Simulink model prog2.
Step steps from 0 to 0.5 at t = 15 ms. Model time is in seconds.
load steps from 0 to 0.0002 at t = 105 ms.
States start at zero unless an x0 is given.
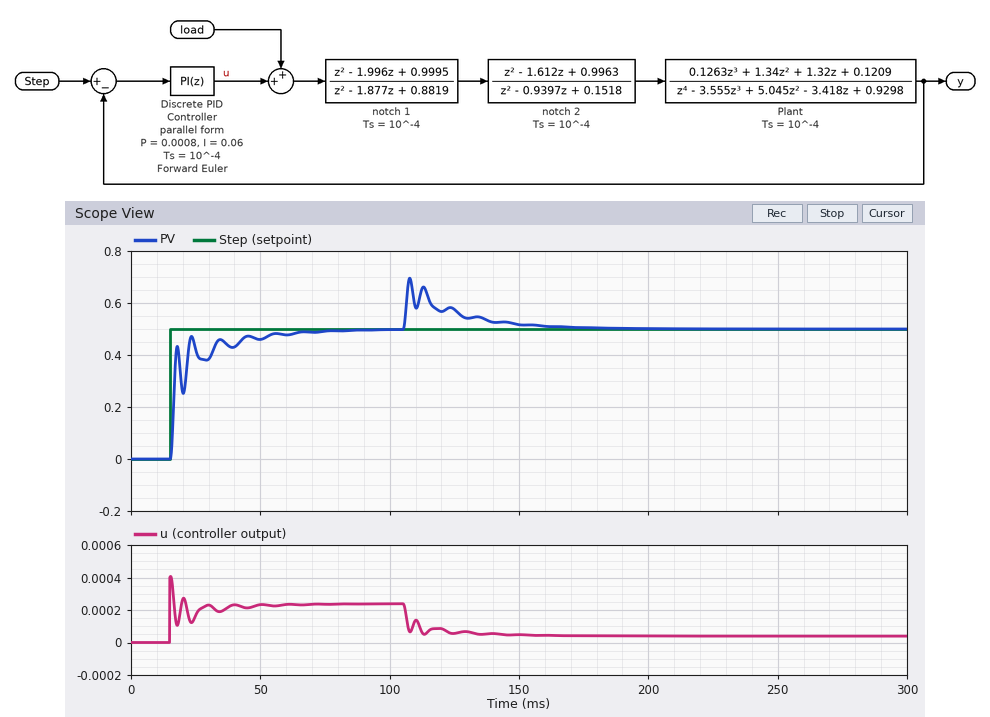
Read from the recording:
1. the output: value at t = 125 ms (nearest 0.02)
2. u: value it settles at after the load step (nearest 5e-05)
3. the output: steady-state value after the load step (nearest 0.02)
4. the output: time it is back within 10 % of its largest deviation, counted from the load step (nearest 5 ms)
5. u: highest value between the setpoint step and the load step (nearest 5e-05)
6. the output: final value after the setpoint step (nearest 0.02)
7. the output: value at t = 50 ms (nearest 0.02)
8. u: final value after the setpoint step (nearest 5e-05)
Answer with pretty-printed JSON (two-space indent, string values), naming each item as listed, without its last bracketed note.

{
  "the output: value at t = 125 ms": "0.58",
  "u: value it settles at after the load step": "0.00005",
  "the output: steady-state value after the load step": "0.50",
  "the output: time it is back within 10 % of its largest deviation, counted from the load step": "45 ms",
  "u: highest value between the setpoint step and the load step": "0.00040",
  "the output: final value after the setpoint step": "0.50",
  "the output: value at t = 50 ms": "0.46",
  "u: final value after the setpoint step": "0.00025"
}
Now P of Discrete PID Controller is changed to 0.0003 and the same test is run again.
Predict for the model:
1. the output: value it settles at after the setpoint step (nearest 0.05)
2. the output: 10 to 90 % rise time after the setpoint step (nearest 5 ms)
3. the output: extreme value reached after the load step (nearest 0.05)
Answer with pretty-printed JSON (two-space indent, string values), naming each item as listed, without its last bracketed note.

{
  "the output: value it settles at after the setpoint step": "0.50",
  "the output: 10 to 90 % rise time after the setpoint step": "15 ms",
  "the output: extreme value reached after the load step": "0.75"
}
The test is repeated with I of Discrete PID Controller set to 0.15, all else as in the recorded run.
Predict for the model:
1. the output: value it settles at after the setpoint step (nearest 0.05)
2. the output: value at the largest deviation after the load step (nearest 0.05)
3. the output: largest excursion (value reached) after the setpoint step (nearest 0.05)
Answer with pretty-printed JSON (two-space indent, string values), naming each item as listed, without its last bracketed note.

{
  "the output: value it settles at after the setpoint step": "0.50",
  "the output: value at the largest deviation after the load step": "0.70",
  "the output: largest excursion (value reached) after the setpoint step": "0.55"
}
